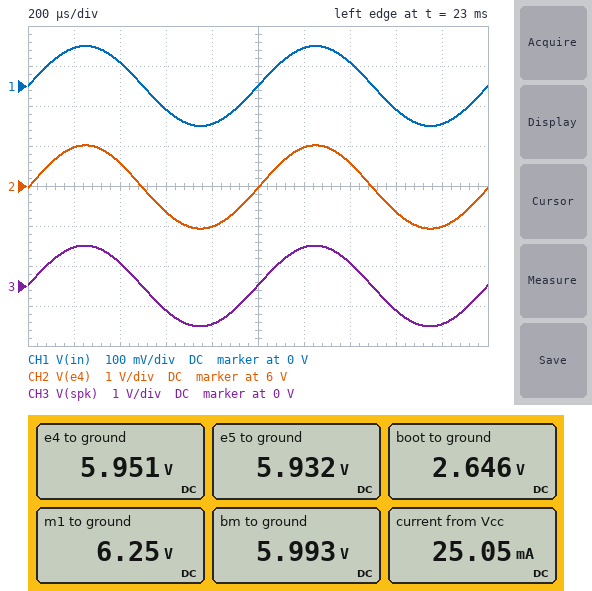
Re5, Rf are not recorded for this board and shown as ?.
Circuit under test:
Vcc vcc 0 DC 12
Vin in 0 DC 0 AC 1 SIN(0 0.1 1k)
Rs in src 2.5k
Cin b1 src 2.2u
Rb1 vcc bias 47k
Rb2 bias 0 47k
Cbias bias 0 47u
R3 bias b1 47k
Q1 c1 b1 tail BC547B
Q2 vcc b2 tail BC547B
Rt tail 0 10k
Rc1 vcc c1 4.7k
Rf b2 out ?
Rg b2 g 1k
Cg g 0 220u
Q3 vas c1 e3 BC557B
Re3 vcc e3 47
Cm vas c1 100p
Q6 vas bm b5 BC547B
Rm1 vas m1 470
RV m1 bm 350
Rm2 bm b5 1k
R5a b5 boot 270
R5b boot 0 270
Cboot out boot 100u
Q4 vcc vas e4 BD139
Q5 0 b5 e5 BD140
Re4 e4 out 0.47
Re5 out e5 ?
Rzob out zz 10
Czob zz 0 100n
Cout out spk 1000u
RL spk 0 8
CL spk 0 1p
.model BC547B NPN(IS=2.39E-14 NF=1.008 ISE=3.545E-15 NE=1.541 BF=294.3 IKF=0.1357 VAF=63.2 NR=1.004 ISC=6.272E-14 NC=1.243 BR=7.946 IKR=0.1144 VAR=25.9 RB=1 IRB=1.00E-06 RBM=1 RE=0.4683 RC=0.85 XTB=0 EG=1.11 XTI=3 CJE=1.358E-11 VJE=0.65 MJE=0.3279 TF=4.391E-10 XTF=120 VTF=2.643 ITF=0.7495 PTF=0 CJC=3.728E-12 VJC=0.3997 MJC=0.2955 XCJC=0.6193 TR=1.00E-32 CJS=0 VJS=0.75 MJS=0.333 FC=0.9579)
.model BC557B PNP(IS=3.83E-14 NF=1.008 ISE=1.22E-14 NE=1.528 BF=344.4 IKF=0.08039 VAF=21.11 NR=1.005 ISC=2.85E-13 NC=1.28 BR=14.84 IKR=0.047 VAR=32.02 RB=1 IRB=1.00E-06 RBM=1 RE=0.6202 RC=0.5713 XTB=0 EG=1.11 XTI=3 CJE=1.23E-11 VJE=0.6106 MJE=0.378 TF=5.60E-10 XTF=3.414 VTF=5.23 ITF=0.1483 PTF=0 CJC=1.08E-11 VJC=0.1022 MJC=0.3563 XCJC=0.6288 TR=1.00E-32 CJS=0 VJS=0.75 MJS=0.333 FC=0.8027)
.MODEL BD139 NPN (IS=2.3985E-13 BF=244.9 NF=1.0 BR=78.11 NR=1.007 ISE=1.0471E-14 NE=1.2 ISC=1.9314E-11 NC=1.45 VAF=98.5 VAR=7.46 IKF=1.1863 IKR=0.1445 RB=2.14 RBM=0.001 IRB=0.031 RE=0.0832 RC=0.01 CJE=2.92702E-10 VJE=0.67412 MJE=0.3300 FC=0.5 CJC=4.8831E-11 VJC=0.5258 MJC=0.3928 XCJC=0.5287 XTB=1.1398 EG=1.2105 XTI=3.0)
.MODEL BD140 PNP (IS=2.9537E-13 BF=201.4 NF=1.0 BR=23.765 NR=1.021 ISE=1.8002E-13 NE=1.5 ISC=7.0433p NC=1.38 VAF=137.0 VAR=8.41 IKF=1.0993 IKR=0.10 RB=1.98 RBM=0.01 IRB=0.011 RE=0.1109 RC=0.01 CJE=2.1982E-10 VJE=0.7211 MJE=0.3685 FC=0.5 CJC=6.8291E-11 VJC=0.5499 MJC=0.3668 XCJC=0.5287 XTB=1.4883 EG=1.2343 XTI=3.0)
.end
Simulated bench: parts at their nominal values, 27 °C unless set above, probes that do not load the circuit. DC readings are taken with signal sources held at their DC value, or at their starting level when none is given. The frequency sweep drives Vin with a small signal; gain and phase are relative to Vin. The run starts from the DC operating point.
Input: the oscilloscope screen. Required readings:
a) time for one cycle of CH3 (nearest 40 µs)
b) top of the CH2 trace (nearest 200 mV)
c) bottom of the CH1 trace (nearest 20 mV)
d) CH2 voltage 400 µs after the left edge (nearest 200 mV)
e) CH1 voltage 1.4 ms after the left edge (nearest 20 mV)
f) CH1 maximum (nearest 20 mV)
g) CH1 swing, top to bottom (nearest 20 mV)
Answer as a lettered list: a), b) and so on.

a) 1.00 ms
b) 7.0 V
c) -100 mV
d) 6.6 V
e) 60 mV
f) 100 mV
g) 200 mV
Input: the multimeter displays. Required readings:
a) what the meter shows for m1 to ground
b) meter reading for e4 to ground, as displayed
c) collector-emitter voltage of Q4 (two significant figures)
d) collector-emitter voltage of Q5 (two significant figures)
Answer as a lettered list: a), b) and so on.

a) 6.25 V
b) 5.951 V
c) 6.0 V
d) -5.9 V
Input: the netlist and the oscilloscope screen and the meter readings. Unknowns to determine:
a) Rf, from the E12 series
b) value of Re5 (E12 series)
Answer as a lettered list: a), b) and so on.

a) 10 kΩ
b) 0.82 Ω
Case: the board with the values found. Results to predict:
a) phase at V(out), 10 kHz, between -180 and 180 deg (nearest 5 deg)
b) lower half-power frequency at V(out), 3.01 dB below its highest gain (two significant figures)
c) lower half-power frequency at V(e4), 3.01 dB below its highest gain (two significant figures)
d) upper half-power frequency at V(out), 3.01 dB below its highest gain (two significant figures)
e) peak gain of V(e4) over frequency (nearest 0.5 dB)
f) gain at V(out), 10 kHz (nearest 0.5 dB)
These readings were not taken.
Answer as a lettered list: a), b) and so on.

a) 0 deg
b) 1.9 Hz
c) 2.0 Hz
d) 600 kHz
e) 20.5 dB
f) 20.0 dB
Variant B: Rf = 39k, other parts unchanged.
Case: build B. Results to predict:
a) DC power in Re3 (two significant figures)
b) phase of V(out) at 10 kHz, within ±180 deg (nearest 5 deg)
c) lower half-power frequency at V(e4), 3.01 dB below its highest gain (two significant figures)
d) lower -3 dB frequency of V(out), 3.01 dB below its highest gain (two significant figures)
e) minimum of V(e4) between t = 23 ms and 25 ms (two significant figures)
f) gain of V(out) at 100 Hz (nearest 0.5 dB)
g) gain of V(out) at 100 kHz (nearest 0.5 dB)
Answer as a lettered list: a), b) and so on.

a) 4.6 mW
b) -5 deg
c) 2.3 Hz
d) 2.2 Hz
e) 2.7 V
f) 30.5 dB
g) 29.0 dB
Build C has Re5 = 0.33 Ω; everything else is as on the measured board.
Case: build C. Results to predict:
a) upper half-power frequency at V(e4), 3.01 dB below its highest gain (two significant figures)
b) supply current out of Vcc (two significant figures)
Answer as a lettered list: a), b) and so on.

a) 650 kHz
b) 27 mA
